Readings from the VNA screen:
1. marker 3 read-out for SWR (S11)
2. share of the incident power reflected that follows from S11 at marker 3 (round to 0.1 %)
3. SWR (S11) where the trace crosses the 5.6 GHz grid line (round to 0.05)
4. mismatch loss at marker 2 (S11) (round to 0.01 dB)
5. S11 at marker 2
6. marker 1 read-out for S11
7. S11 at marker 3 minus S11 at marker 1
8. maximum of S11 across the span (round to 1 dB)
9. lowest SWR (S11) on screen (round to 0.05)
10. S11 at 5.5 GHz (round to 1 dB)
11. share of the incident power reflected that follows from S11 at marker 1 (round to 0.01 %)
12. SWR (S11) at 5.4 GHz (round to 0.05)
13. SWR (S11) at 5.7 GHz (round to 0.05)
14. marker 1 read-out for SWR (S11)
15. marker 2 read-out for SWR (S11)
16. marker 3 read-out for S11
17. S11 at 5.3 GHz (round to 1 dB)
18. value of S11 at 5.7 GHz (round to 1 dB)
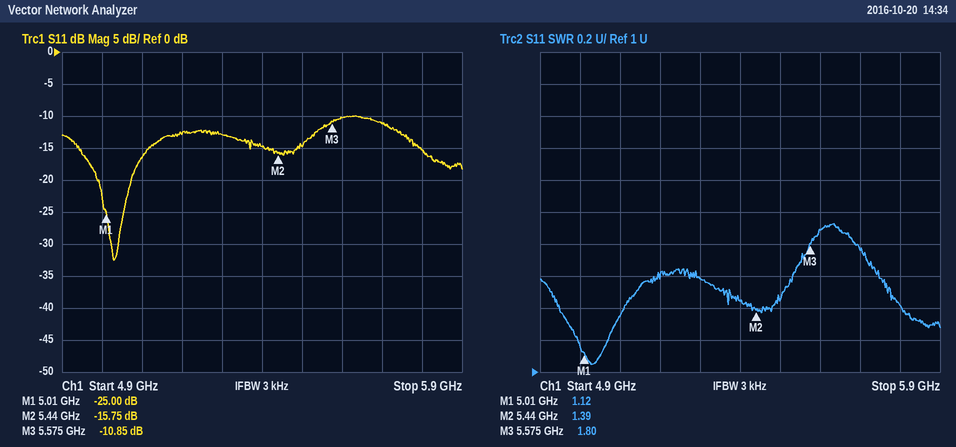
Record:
1.80
8.2 %
1.90
0.12 dB
-15.75 dB
-25.00 dB
14.15 dB
-10 dB
1.05
-15 dB
0.32 %
1.45
1.75
1.12
1.39
-10.85 dB
-13 dB
-11 dB
